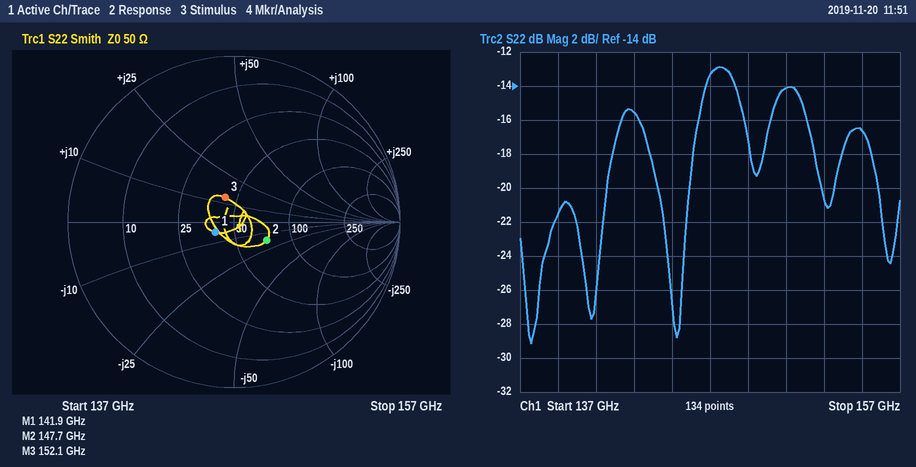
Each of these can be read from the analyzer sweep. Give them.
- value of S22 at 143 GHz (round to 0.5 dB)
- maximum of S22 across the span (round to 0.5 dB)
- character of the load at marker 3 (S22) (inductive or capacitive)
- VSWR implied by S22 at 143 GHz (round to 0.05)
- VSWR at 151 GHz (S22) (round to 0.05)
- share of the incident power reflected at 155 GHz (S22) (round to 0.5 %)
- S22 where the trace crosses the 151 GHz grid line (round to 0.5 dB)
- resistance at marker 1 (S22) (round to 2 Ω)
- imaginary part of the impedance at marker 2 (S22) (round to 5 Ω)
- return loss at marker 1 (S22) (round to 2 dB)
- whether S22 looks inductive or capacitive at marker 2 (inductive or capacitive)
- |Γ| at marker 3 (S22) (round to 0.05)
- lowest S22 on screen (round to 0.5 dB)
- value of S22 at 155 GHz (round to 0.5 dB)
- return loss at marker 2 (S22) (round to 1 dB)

-15.5 dB
-13.0 dB
inductive
1.40
1.50
2.0 %
-14.0 dB
40 Ω
-15 Ω
18 dB
capacitive
0.15
-29.0 dB
-16.5 dB
13 dB
